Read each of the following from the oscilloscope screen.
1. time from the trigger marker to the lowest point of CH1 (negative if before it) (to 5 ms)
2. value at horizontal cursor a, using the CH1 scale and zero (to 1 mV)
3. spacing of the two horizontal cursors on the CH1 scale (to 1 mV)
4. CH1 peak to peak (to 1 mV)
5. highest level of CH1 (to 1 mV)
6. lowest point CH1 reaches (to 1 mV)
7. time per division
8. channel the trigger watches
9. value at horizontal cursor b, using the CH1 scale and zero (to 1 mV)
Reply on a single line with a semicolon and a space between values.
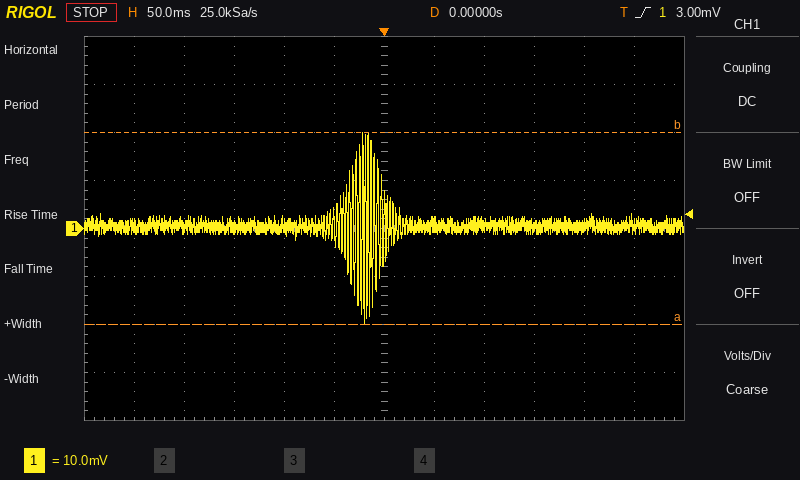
-20 ms; -20 mV; 40 mV; 40 mV; 20 mV; -20 mV; 50 ms; CH1; 20 mV
